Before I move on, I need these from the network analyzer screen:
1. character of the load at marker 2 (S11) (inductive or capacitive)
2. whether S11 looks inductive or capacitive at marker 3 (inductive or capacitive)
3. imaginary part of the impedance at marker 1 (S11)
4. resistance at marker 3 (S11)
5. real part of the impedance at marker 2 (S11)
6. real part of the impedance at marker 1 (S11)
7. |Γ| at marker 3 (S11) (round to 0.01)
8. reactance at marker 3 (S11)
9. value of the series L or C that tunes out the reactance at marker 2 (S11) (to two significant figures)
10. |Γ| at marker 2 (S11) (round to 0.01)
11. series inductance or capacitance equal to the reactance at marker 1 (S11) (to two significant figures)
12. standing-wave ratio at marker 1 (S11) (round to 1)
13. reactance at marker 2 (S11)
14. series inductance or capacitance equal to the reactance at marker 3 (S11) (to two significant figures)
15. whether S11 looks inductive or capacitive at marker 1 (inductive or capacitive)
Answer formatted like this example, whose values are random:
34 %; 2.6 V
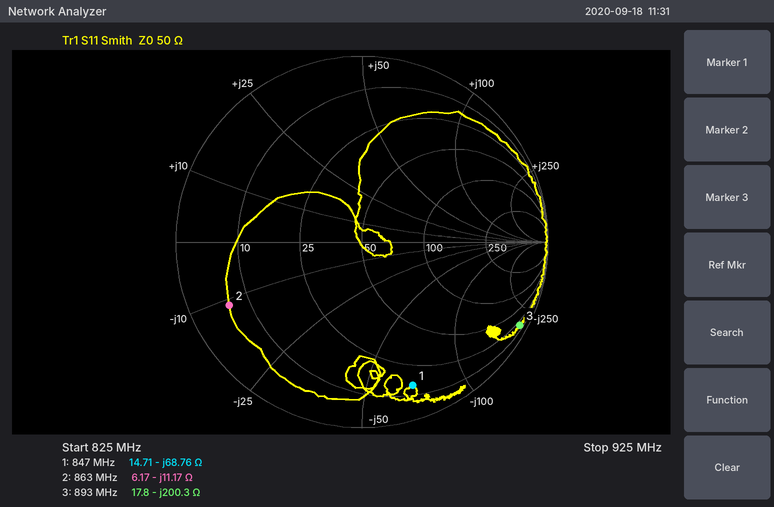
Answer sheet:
capacitive; capacitive; -68.76 Ω; 17.8 Ω; 6.17 Ω; 14.71 Ω; 0.96; -200.3 Ω; 2.1 nH; 0.79; 2.7 pF; 10; -11.17 Ω; 890 fF; capacitive
